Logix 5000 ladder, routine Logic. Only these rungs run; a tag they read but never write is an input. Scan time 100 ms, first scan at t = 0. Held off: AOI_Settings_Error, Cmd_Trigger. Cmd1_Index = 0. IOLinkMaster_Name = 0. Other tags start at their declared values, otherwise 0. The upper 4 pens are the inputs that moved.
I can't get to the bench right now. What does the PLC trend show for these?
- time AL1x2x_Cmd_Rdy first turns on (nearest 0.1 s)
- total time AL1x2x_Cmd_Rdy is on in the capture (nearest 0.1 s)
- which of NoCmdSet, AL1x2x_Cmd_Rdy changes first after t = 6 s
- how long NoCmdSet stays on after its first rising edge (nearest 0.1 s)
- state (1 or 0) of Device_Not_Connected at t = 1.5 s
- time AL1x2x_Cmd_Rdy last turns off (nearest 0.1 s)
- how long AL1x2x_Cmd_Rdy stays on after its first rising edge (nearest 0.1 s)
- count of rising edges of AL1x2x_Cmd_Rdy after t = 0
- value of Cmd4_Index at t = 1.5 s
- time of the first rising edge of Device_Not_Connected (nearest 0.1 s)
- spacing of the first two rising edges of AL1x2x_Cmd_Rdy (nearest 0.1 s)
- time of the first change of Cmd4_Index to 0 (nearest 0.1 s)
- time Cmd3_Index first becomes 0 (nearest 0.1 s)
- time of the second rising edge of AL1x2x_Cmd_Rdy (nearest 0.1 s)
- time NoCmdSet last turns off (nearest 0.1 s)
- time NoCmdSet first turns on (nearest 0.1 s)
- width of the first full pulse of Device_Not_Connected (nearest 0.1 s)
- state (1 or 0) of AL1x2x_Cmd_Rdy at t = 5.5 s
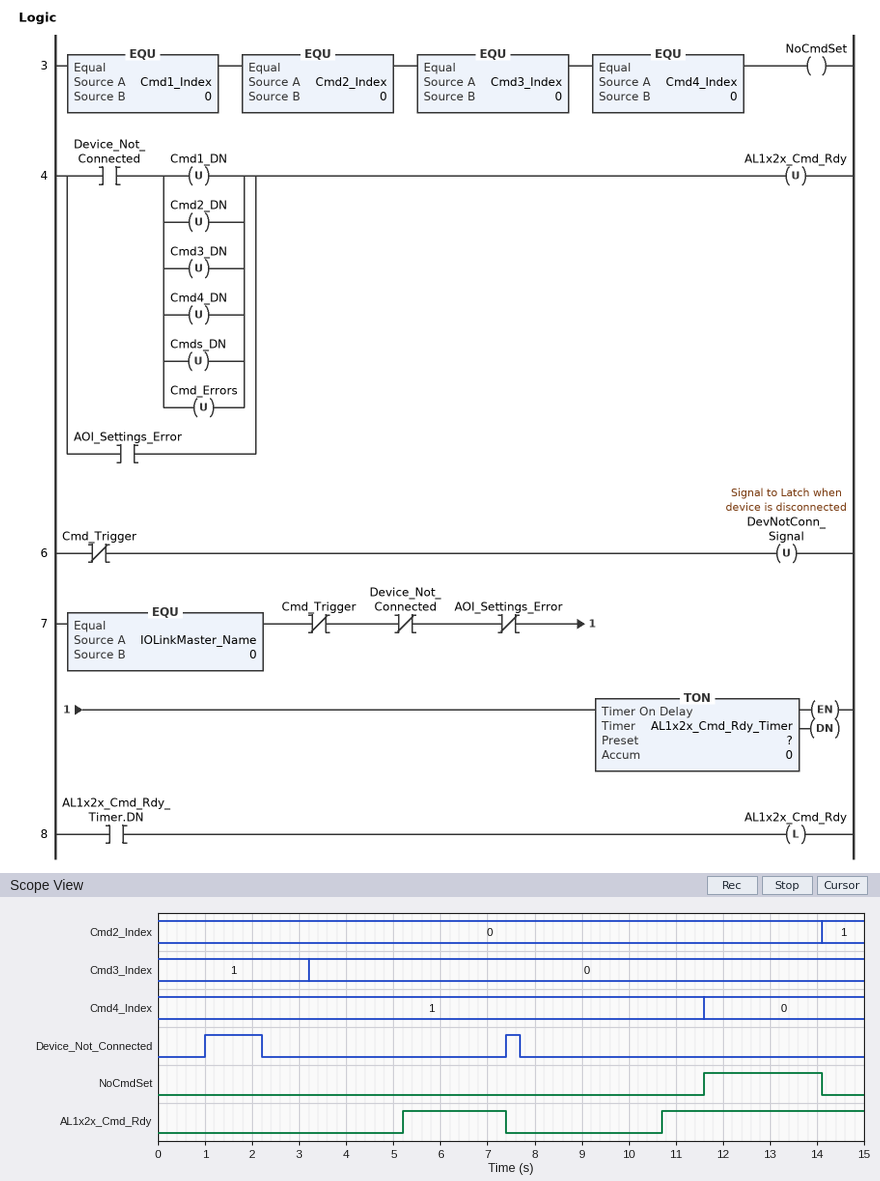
5.2 s
6.5 s
AL1x2x_Cmd_Rdy
2.5 s
1
7.4 s
2.2 s
2
1
1.0 s
5.5 s
11.6 s
3.2 s
10.7 s
14.1 s
11.6 s
1.2 s
1
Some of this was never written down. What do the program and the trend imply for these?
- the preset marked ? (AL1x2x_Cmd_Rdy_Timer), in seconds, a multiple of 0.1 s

3.0 s
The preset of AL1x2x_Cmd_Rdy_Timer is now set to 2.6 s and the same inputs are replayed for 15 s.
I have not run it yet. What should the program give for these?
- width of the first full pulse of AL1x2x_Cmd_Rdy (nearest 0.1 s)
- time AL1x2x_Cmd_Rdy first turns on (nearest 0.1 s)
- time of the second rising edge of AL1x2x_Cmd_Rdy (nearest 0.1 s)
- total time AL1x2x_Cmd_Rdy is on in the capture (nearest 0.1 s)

2.6 s
4.8 s
10.3 s
7.3 s
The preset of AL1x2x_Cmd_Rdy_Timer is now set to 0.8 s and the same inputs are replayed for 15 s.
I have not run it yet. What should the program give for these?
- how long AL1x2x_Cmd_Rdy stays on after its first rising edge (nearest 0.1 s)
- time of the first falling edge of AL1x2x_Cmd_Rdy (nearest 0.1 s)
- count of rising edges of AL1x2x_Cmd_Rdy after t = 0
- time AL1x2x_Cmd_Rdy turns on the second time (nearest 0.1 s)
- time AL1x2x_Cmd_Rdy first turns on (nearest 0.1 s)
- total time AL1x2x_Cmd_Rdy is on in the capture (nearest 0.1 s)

0.2 s
1.0 s
3
3.0 s
0.8 s
11.1 s
